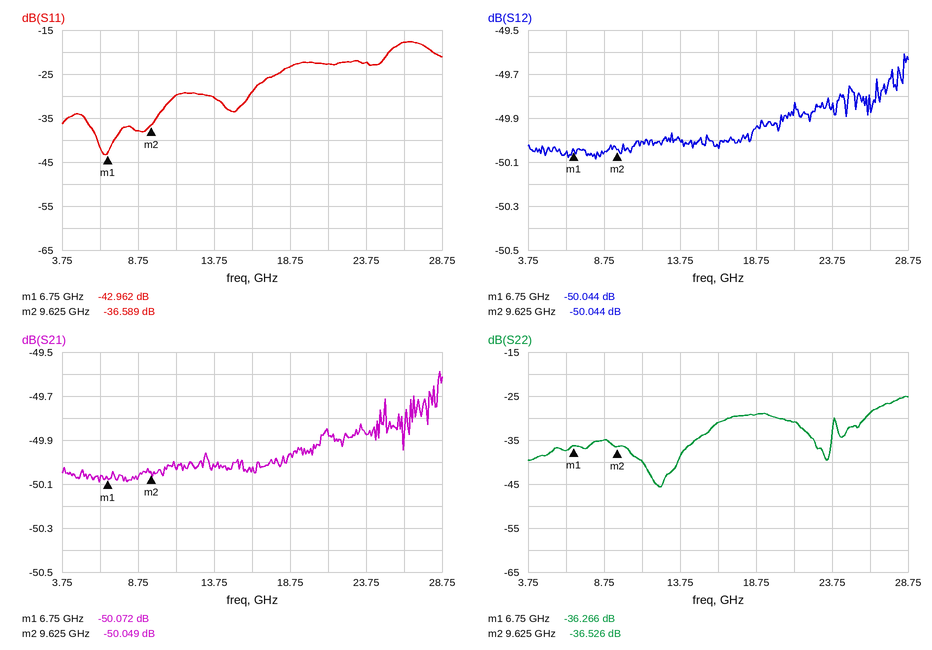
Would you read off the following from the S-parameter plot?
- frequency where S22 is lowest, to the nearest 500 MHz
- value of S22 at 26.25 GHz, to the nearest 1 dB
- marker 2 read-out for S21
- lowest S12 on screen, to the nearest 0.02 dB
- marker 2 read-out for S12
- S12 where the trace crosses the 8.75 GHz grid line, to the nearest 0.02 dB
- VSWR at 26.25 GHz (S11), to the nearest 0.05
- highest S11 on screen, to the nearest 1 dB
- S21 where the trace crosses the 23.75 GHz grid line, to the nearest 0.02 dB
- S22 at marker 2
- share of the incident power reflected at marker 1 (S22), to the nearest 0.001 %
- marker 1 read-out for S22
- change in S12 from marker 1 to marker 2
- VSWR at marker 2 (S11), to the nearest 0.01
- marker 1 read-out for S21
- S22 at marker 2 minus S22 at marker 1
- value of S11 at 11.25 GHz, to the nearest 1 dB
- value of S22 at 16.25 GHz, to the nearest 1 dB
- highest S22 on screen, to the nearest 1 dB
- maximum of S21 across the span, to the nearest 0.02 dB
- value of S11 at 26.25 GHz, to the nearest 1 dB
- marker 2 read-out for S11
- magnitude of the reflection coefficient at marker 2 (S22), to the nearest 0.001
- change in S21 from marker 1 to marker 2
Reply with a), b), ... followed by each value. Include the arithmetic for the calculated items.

a) 12.5 GHz
b) -29 dB
c) -50.049 dB
d) -50.08 dB
e) -50.044 dB
f) -50.06 dB
g) |Γ| = 10^(-18/20) = 0.1259; VSWR = (1 + 0.1259)/(1 − 0.1259) ≈ 1.29, so 1.30 to the nearest 0.05
h) -18 dB
i) -49.88 dB
j) -36.526 dB
k) 10^(-36.266/10) ≈ 0.024 %
l) -36.266 dB
m) -50.044 − (-50.044) = 0.000 dB
n) (1 + 0.0148)/(1 − 0.0148) ≈ 1.03
o) -50.072 dB
p) -36.526 − (-36.266) = -0.260 dB
q) -30 dB
r) -31 dB
s) -25 dB
t) -49.58 dB
u) -18 dB
v) -36.589 dB
w) 10^(-36.526/20) ≈ 0.015
x) -50.049 − (-50.072) = 0.023 dB
